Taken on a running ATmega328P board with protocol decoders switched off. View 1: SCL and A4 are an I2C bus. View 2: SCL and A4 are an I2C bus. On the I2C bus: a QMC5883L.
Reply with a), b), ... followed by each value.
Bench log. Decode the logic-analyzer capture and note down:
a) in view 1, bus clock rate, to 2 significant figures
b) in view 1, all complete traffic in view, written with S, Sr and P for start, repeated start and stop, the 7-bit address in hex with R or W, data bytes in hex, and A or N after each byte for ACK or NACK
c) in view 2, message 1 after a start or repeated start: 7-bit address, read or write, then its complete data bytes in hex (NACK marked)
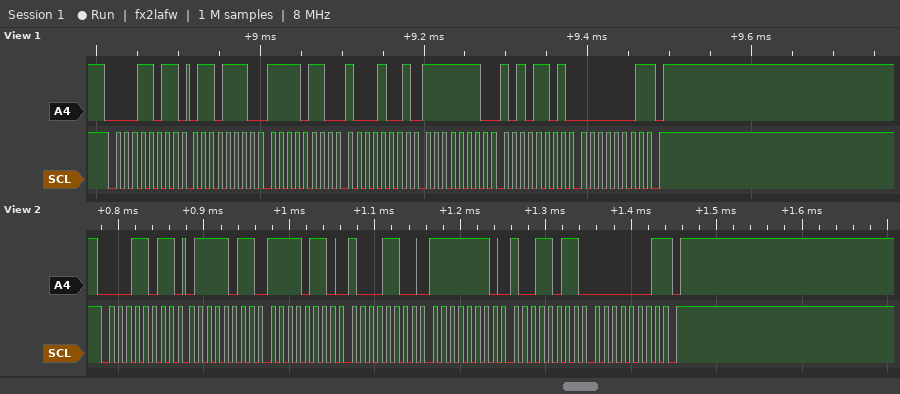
a) 100 kHz
b) S 0DR A 6E A F6 A 89 A FE A AD A 01 N P
c) 0x0D read: 7B F6 8C FE 9B 01 NACK
